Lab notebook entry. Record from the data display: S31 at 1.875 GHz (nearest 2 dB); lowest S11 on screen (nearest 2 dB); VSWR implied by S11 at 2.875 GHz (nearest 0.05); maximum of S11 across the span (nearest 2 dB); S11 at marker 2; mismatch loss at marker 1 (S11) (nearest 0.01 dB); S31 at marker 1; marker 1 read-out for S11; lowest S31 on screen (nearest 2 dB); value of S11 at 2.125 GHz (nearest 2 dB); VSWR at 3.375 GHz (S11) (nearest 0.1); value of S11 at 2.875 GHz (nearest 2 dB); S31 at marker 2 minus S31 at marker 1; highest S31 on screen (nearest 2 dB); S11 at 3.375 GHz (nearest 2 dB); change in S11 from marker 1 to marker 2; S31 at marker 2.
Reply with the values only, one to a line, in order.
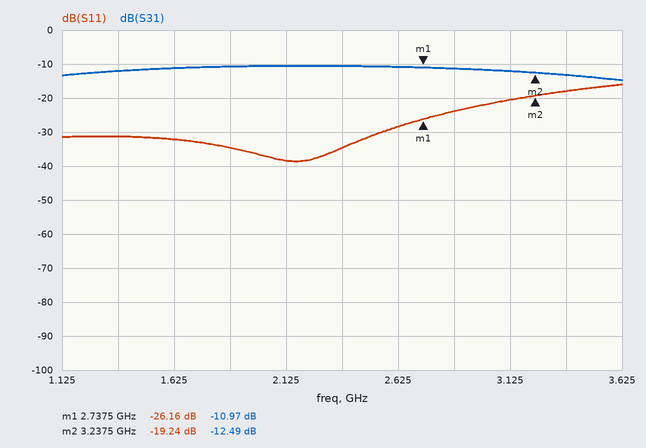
-10 dB
-38 dB
1.15
-16 dB
-19.24 dB
0.01 dB
-10.97 dB
-26.16 dB
-14 dB
-38 dB
1.3
-24 dB
-1.52 dB
-10 dB
-18 dB
6.92 dB
-12.49 dB
